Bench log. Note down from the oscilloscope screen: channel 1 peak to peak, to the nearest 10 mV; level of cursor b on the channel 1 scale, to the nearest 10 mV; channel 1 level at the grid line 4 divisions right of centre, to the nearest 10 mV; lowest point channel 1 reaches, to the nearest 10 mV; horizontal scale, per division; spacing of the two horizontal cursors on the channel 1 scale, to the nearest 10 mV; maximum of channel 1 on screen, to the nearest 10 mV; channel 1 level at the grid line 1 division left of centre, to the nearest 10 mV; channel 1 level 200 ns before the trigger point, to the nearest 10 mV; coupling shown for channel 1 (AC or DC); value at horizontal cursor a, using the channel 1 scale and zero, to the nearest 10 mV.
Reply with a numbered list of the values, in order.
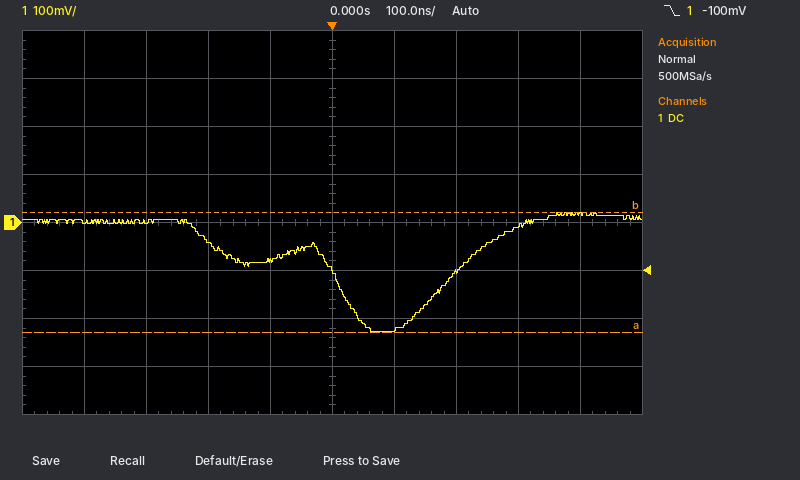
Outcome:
1. 250 mV
2. 20 mV
3. 20 mV
4. -230 mV
5. 100 ns
6. 250 mV
7. 20 mV
8. -80 mV
9. -40 mV
10. DC
11. -230 mV
